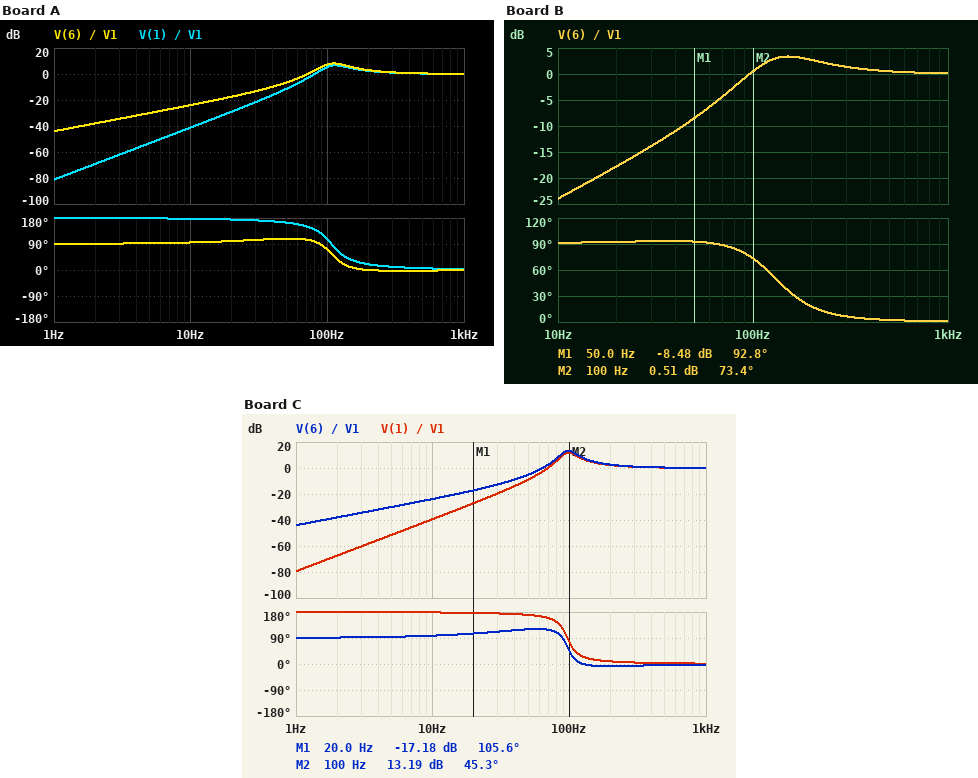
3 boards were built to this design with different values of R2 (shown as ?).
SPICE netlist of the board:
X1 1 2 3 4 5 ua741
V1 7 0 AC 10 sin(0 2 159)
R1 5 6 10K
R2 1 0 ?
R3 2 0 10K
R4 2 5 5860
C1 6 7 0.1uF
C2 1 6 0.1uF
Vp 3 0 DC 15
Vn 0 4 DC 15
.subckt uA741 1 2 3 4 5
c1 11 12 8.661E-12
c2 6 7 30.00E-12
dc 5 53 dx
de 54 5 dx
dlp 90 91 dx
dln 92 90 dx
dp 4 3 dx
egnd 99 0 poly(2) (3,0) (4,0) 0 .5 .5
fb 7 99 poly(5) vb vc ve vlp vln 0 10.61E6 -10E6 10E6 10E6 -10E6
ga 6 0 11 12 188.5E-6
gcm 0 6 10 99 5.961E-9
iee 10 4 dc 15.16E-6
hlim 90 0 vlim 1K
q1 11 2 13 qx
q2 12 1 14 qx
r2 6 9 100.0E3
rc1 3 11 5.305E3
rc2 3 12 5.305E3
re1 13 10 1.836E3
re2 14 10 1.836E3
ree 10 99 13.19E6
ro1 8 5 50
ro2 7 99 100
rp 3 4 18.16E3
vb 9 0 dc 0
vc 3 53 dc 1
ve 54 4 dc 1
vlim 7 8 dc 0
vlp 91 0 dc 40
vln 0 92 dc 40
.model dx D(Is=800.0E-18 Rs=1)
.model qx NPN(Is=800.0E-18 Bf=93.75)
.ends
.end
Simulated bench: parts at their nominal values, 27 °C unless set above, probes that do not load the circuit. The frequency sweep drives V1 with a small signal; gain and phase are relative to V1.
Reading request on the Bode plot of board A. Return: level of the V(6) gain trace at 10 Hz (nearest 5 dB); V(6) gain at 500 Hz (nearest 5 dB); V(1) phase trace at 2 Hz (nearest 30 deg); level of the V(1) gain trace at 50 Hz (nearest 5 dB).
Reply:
-25 dB
0 dB
180 deg
-10 dB
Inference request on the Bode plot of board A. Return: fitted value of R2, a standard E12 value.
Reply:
22 kΩ
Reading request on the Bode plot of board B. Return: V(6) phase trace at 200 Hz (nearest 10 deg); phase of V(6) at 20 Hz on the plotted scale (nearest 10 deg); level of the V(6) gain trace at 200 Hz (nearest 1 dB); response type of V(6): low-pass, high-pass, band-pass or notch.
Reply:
20 deg
90 deg
3 dB
high-pass
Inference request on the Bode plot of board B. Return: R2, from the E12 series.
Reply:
15 kΩ
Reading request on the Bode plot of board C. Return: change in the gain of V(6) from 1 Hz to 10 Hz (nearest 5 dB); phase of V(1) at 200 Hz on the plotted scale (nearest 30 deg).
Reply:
20 dB
0 deg
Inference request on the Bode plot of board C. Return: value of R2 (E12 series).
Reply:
27 kΩ
